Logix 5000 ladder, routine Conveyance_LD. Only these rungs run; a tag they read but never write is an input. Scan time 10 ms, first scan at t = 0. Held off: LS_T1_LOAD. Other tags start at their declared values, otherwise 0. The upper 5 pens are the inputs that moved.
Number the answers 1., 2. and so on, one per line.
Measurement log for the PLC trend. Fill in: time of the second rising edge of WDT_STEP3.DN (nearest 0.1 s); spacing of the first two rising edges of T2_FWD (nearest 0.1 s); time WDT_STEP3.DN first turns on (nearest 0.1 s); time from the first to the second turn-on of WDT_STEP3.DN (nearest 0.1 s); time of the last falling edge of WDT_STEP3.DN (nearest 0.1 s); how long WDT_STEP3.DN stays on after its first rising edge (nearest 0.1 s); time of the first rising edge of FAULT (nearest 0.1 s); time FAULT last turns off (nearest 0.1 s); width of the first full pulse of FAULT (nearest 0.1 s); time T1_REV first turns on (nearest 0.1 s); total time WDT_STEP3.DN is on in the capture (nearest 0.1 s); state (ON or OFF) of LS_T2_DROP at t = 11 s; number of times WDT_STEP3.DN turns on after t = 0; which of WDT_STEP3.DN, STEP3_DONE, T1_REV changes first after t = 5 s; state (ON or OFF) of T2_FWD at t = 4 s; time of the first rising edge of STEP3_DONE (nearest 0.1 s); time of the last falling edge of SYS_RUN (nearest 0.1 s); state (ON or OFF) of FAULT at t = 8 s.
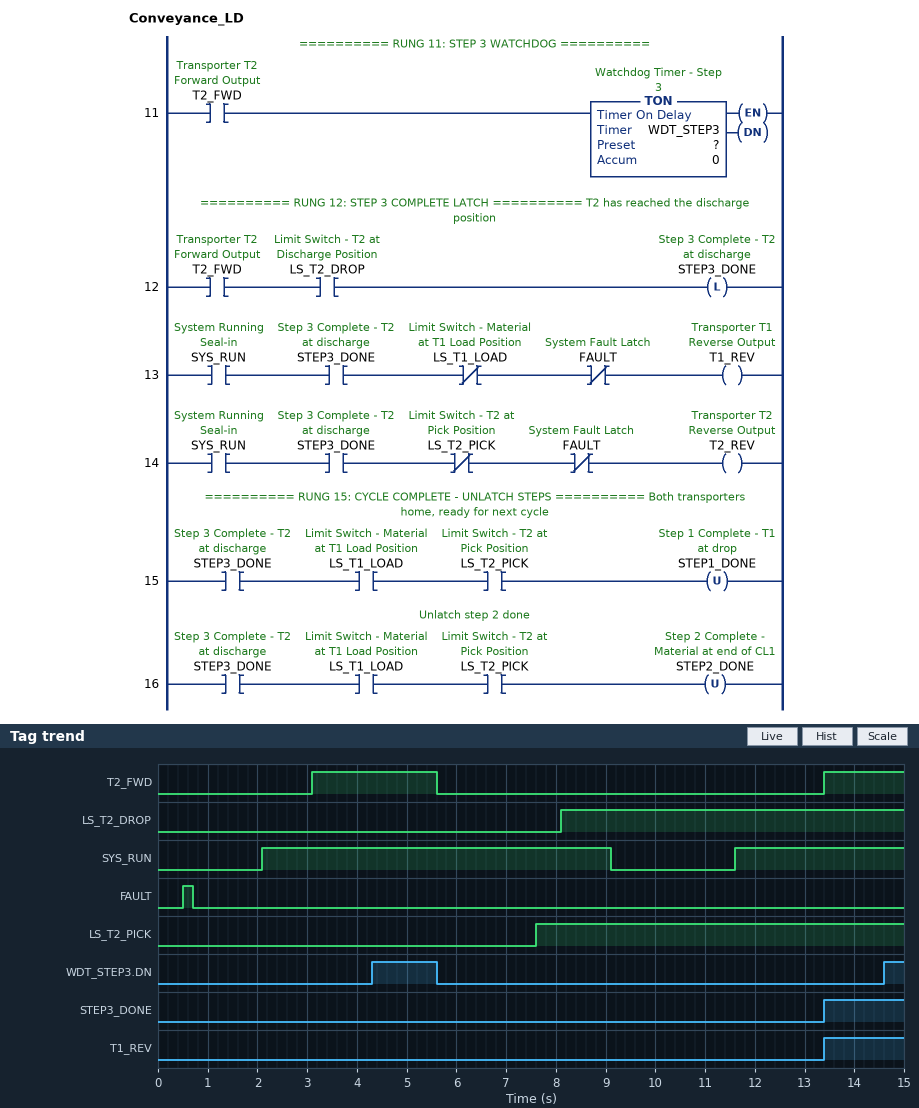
1. 14.6 s
2. 10.3 s
3. 4.3 s
4. 10.3 s
5. 5.6 s
6. 1.3 s
7. 0.5 s
8. 0.7 s
9. 0.2 s
10. 13.4 s
11. 1.7 s
12. ON
13. 2
14. WDT_STEP3.DN
15. ON
16. 13.4 s
17. 9.1 s
18. OFF
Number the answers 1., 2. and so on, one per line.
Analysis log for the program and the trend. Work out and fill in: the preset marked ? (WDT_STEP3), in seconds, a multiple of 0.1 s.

1. 1.2 s
